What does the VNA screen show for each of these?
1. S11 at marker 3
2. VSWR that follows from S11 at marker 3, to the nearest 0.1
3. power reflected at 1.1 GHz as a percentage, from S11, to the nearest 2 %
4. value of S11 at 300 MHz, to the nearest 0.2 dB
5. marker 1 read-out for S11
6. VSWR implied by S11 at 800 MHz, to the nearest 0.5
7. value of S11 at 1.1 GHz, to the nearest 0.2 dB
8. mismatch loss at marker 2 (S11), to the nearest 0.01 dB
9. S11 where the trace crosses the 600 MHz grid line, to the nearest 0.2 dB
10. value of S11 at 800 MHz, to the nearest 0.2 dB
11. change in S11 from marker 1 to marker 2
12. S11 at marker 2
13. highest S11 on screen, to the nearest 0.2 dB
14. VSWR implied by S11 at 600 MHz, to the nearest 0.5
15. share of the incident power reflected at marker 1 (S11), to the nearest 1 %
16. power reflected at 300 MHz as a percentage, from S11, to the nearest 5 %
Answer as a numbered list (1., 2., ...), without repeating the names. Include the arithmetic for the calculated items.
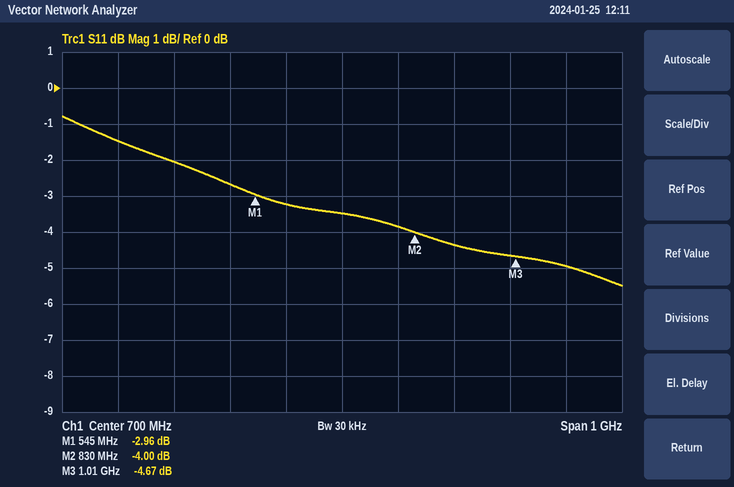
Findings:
1. -4.67 dB
2. (1 + 0.5841)/(1 − 0.5841) ≈ 3.8
3. 10^(-5/10) ≈ 32 %
4. -1.4 dB
5. -2.96 dB
6. |Γ| = 10^(-3.8/20) = 0.6457; VSWR = (1 + 0.6457)/(1 − 0.6457) ≈ 4.64, so 4.5 to the nearest 0.5
7. -5.0 dB
8. −10 log10(1 − 10^(-4/10)) ≈ 2.20 dB
9. -3.2 dB
10. -3.8 dB
11. -4 − (-2.96) = -1.04 dB
12. -4.00 dB
13. -0.8 dB
14. |Γ| = 10^(-3.2/20) = 0.6918; VSWR = (1 + 0.6918)/(1 − 0.6918) ≈ 5.5
15. 10^(-2.96/10) ≈ 51 %
16. 10^(-1.4/10) ≈ 72.4 %, so 70 % to the nearest 5 %
